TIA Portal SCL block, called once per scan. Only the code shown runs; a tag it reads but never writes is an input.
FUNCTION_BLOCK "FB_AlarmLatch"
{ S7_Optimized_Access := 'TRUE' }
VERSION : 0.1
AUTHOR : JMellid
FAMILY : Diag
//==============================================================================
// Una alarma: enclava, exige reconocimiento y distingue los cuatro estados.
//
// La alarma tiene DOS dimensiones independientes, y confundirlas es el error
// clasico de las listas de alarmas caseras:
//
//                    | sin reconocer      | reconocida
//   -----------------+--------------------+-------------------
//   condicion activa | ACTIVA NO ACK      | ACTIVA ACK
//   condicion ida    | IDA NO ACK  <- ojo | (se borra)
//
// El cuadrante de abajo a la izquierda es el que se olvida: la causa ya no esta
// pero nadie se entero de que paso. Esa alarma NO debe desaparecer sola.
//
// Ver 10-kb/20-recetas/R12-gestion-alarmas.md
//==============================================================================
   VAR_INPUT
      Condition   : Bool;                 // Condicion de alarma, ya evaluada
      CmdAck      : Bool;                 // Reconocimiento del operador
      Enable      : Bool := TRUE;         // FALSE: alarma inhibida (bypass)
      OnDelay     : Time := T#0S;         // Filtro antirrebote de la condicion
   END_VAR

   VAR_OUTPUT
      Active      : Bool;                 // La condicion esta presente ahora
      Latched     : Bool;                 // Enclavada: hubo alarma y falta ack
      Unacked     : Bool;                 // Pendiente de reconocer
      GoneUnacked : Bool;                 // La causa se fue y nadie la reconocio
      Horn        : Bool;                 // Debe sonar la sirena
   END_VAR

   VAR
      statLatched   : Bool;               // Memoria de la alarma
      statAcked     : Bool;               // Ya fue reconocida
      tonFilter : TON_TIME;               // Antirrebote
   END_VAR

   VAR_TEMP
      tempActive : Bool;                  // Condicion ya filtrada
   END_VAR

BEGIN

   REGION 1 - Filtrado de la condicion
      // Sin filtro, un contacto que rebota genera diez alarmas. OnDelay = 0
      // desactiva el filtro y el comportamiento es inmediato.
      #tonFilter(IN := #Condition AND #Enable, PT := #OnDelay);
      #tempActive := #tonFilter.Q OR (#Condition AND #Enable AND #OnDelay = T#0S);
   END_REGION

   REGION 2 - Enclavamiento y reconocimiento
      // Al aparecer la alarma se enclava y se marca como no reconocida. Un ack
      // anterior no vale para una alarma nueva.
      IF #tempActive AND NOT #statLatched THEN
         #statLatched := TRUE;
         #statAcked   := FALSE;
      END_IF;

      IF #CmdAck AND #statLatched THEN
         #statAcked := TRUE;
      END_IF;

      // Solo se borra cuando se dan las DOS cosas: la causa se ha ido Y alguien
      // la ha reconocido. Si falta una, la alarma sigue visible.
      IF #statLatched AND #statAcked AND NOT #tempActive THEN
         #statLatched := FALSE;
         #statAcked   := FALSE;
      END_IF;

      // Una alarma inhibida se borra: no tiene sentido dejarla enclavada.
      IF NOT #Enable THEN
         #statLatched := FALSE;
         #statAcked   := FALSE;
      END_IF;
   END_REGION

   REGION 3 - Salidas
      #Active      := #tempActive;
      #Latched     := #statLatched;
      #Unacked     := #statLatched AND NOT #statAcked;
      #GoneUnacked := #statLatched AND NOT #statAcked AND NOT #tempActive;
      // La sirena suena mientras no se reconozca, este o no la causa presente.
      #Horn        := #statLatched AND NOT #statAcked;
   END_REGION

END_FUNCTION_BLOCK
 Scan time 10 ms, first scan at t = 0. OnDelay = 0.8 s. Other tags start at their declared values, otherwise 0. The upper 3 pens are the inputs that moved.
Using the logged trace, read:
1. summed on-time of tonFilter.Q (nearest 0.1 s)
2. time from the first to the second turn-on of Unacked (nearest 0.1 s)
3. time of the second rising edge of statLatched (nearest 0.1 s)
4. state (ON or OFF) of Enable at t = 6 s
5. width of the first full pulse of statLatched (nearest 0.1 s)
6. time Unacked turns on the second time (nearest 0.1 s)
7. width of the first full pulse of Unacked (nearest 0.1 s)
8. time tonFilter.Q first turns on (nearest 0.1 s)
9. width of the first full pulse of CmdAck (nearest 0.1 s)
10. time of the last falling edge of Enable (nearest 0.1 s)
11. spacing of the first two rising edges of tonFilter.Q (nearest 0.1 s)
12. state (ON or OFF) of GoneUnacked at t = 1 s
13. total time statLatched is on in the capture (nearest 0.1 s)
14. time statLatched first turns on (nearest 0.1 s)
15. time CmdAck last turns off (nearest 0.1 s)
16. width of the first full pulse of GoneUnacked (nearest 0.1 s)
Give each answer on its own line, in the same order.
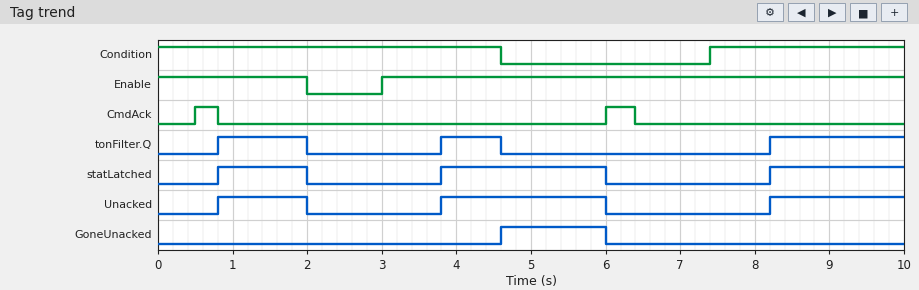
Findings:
3.8 s
3.0 s
3.8 s
ON
1.2 s
3.8 s
1.2 s
0.8 s
0.3 s
2.0 s
3.0 s
OFF
5.2 s
0.8 s
6.4 s
1.4 s
